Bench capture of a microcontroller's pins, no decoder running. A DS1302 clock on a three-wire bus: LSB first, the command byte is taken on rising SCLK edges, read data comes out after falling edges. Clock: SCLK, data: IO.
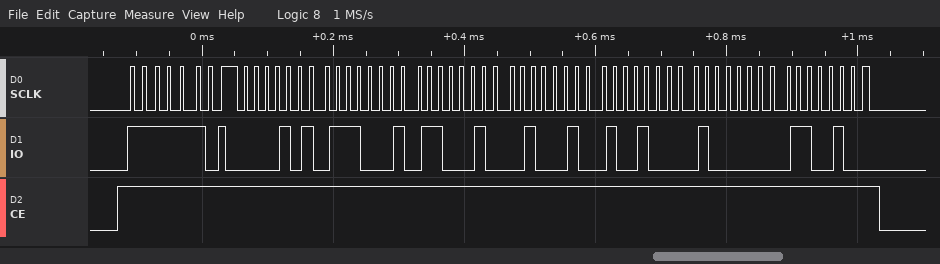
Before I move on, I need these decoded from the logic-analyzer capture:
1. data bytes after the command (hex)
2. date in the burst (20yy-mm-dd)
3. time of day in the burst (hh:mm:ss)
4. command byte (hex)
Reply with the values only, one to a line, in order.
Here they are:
50 47 23 22 09 01 13
2013-09-22
23:47:50
0xBF
